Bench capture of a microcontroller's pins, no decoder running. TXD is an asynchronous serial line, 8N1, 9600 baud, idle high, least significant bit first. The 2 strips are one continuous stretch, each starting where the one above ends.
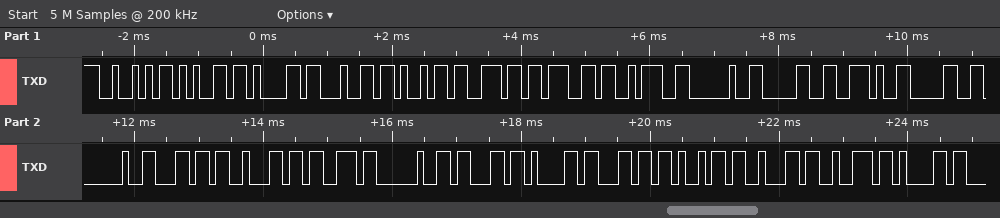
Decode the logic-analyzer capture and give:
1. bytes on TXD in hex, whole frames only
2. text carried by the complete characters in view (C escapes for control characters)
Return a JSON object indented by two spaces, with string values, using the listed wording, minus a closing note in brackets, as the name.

{
  "bytes on TXD in hex, whole frames only": "52 65 61 64 69 6E 67 3A 20 30 2E 30 20 6C 62 73 20 63 61 6C 69 62 72 61",
  "text carried by the complete characters in view": "\"Reading: 0.0 lbs calibra\""
}
